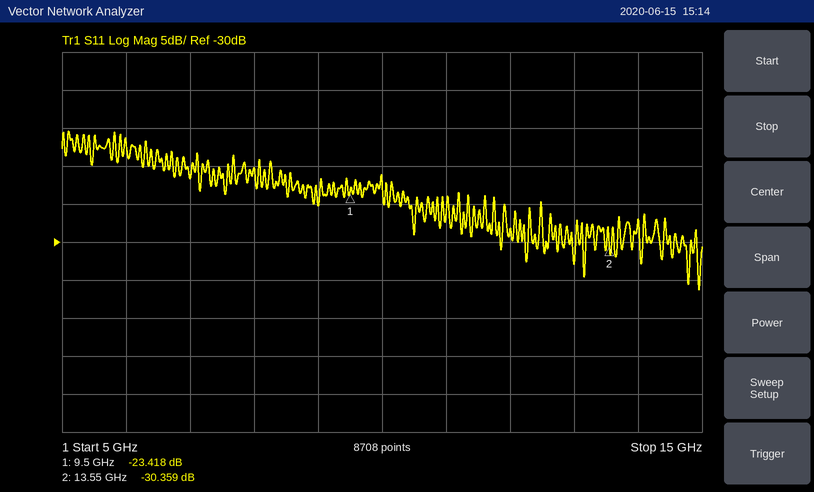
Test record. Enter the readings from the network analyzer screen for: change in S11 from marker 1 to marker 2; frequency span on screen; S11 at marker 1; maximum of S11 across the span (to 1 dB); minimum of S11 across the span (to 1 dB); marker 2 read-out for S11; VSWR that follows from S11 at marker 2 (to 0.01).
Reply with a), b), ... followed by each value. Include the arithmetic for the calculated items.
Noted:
a) -30.359 − (-23.418) = -6.941 dB
b) 10 GHz
c) -23.418 dB
d) -15 dB
e) -36 dB
f) -30.359 dB
g) (1 + 0.0303)/(1 − 0.0303) ≈ 1.06
